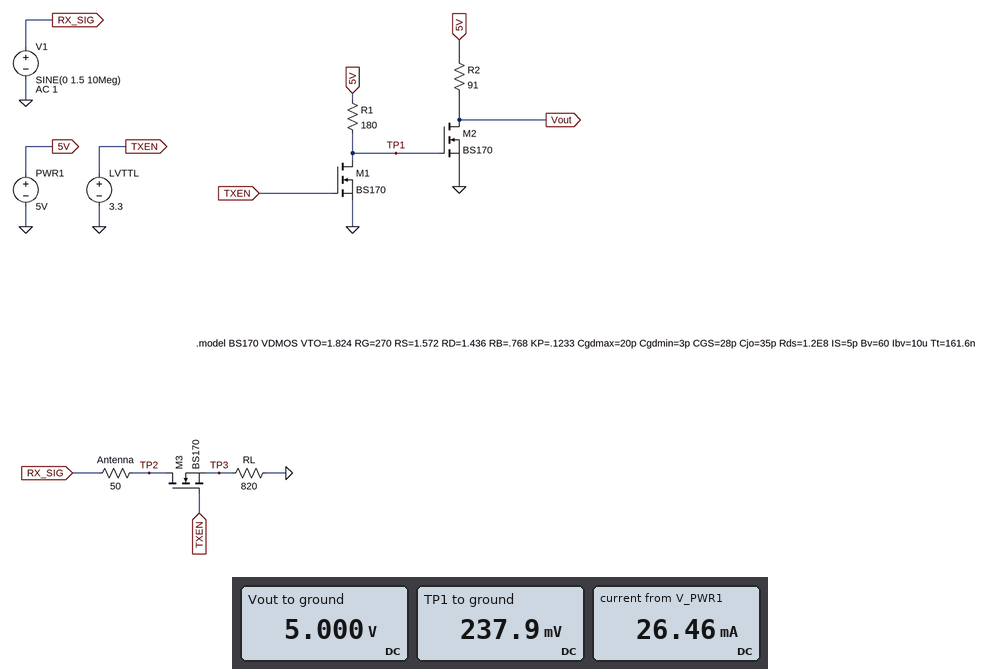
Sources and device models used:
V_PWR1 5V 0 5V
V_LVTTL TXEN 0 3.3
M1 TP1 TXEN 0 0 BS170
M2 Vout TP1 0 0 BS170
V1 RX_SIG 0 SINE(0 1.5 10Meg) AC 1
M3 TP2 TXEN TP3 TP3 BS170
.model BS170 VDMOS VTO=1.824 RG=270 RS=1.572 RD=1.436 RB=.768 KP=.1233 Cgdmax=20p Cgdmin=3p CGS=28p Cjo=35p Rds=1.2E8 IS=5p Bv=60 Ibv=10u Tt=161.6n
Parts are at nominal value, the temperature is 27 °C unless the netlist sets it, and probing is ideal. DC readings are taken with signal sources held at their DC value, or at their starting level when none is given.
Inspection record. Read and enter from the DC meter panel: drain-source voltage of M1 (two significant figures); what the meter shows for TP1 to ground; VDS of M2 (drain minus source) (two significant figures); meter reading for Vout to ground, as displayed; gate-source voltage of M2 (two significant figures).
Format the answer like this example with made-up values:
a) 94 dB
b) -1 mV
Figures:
a) 240 mV
b) 237.9 mV
c) 5.0 V
d) 5.000 V
e) 240 mV
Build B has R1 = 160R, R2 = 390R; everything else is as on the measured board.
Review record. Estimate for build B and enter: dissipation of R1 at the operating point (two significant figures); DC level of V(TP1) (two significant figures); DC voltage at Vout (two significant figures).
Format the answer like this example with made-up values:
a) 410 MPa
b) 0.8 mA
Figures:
a) 140 mW
b) 270 mV
c) 5.0 V
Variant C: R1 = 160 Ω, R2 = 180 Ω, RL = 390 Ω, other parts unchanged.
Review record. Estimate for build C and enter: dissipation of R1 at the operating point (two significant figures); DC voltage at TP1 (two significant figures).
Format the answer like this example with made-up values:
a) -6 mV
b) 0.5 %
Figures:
a) 140 mW
b) 270 mV
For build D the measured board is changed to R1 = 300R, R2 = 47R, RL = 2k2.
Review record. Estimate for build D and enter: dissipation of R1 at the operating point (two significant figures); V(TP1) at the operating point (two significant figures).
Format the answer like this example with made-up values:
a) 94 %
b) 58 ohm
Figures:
a) 79 mW
b) 140 mV
